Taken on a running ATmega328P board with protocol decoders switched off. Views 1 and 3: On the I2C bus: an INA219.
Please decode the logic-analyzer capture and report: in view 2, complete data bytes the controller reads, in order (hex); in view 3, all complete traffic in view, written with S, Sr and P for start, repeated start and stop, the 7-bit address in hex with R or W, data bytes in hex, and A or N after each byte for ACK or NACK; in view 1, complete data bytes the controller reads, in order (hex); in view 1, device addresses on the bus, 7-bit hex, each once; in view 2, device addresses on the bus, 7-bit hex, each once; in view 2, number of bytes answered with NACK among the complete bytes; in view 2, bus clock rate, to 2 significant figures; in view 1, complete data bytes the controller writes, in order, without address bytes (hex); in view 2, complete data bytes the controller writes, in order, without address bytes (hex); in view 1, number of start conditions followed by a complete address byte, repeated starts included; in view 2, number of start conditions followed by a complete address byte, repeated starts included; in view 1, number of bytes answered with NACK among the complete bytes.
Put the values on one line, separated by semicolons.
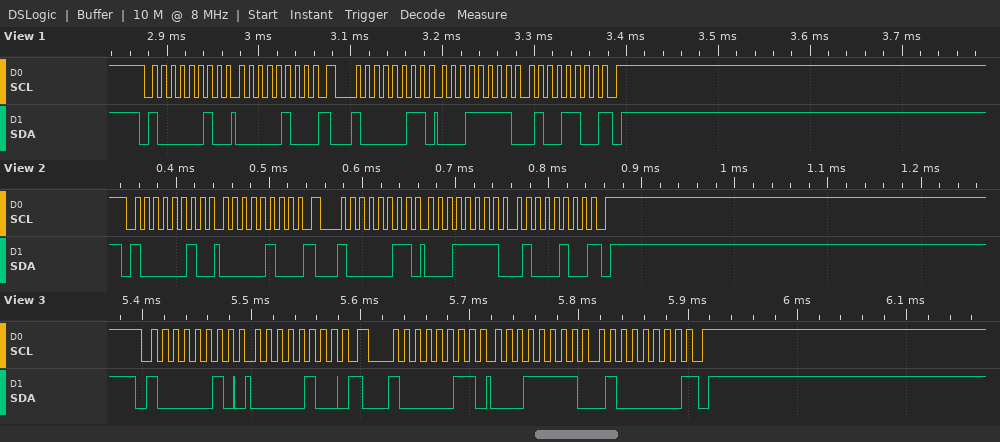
1F 44; S 41W A 04 A Sr 41R A 1F A 40 N P; 1F 4C; 0x41; 0x41; 1; 100 kHz; 04; 04; 2; 2; 1
